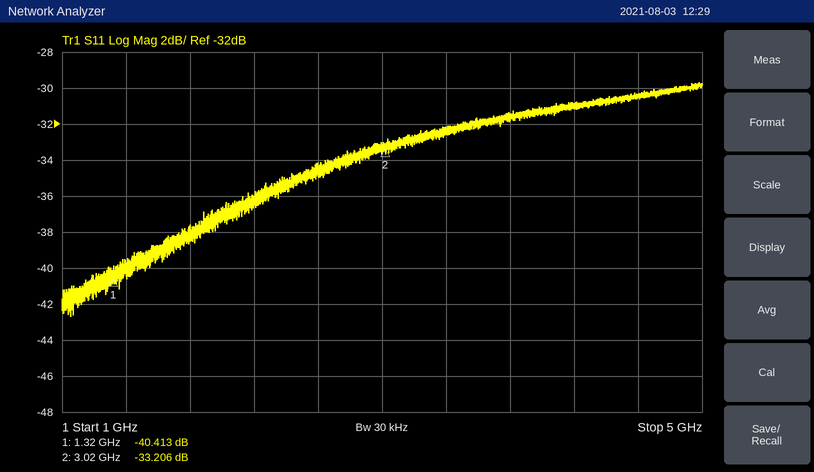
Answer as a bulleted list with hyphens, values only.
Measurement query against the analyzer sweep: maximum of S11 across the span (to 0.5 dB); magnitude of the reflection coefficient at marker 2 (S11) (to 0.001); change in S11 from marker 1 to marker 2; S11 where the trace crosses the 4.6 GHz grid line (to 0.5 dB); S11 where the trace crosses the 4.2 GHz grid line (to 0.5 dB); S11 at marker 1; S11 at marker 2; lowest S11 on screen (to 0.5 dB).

- -29.5 dB
- 0.022
- 7.207 dB
- -30.5 dB
- -31.0 dB
- -40.413 dB
- -33.206 dB
- -42.5 dB
